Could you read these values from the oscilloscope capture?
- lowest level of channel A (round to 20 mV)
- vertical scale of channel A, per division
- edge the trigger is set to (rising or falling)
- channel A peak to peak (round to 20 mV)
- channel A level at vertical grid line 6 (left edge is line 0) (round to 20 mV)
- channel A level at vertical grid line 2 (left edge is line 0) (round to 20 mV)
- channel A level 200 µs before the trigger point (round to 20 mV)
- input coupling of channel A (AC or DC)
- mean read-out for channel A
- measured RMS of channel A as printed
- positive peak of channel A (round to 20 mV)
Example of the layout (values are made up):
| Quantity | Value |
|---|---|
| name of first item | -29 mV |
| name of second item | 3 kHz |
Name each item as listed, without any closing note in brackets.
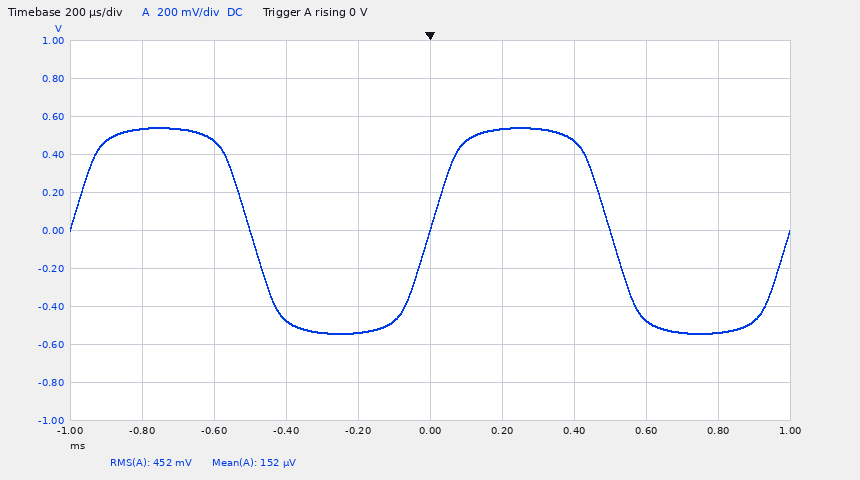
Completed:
| Quantity | Value |
|---|---|
| lowest level of channel A | -540 mV |
| vertical scale of channel A, per division | 200 mV |
| edge the trigger is set to | rising |
| channel A peak to peak | 1.08 V |
| channel A level at vertical grid line 6 (left edge is line 0) | 540 mV |
| channel A level at vertical grid line 2 (left edge is line 0) | 480 mV |
| channel A level 200 µs before the trigger point | -540 mV |
| input coupling of channel A | DC |
| mean read-out for channel A | 152 µV |
| measured RMS of channel A as printed | 452 mV |
| positive peak of channel A | 540 mV |
